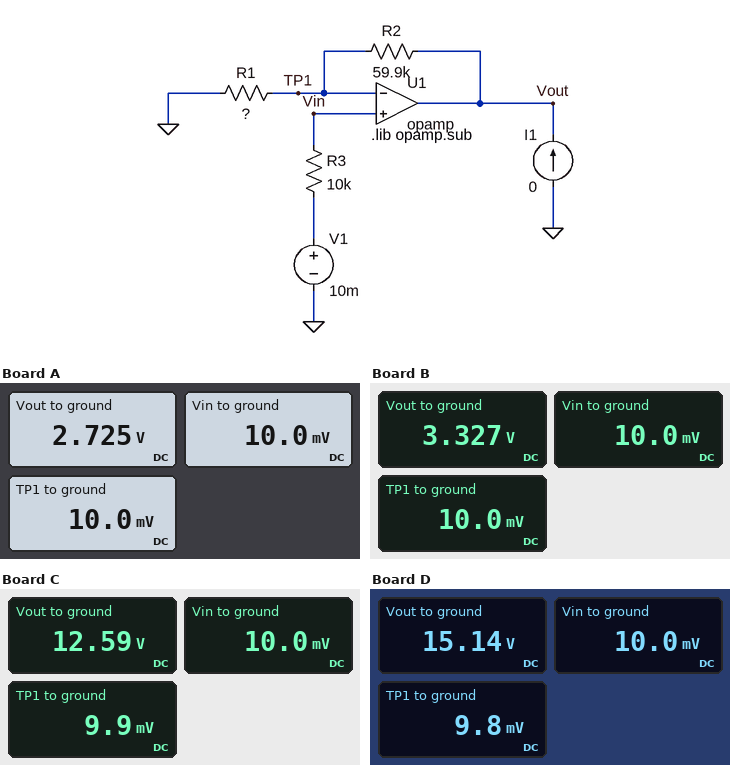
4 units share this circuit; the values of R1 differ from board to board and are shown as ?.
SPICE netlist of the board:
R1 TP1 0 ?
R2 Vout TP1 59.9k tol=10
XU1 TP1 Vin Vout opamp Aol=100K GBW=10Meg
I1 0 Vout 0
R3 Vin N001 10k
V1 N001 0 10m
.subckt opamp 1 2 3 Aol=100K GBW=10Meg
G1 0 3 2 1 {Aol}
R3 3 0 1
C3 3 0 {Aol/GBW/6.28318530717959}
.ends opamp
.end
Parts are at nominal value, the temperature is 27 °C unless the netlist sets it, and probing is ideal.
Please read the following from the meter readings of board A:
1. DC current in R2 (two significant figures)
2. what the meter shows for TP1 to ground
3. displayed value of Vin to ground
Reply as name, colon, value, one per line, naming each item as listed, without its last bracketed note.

DC current in R2: 45 µA
what the meter shows for TP1 to ground: 10.0 mV
displayed value of Vin to ground: 10.0 mV
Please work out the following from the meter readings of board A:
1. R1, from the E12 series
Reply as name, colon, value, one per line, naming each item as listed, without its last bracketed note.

R1, from the E12 series: 220 Ω
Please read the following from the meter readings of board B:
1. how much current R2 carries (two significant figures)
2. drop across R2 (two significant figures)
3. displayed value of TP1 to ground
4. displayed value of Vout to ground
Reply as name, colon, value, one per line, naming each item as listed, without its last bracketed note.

how much current R2 carries: 55 µA
drop across R2: 3.3 V
displayed value of TP1 to ground: 10.0 mV
displayed value of Vout to ground: 3.327 V
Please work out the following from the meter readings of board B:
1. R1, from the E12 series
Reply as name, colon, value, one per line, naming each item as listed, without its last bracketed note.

R1, from the E12 series: 180 Ω
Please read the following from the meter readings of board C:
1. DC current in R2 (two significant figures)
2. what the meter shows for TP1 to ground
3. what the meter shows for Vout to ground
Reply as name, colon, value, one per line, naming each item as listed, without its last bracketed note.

DC current in R2: 210 µA
what the meter shows for TP1 to ground: 9.9 mV
what the meter shows for Vout to ground: 12.59 V
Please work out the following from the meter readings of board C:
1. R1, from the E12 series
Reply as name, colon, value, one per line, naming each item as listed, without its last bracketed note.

R1, from the E12 series: 47 Ω
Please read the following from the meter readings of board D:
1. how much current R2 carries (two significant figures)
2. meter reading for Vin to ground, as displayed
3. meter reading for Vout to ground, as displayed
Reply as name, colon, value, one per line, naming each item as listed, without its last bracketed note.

how much current R2 carries: 250 µA
meter reading for Vin to ground, as displayed: 10.0 mV
meter reading for Vout to ground, as displayed: 15.14 V
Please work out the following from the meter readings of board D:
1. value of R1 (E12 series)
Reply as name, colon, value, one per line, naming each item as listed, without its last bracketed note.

value of R1: 39 Ω
